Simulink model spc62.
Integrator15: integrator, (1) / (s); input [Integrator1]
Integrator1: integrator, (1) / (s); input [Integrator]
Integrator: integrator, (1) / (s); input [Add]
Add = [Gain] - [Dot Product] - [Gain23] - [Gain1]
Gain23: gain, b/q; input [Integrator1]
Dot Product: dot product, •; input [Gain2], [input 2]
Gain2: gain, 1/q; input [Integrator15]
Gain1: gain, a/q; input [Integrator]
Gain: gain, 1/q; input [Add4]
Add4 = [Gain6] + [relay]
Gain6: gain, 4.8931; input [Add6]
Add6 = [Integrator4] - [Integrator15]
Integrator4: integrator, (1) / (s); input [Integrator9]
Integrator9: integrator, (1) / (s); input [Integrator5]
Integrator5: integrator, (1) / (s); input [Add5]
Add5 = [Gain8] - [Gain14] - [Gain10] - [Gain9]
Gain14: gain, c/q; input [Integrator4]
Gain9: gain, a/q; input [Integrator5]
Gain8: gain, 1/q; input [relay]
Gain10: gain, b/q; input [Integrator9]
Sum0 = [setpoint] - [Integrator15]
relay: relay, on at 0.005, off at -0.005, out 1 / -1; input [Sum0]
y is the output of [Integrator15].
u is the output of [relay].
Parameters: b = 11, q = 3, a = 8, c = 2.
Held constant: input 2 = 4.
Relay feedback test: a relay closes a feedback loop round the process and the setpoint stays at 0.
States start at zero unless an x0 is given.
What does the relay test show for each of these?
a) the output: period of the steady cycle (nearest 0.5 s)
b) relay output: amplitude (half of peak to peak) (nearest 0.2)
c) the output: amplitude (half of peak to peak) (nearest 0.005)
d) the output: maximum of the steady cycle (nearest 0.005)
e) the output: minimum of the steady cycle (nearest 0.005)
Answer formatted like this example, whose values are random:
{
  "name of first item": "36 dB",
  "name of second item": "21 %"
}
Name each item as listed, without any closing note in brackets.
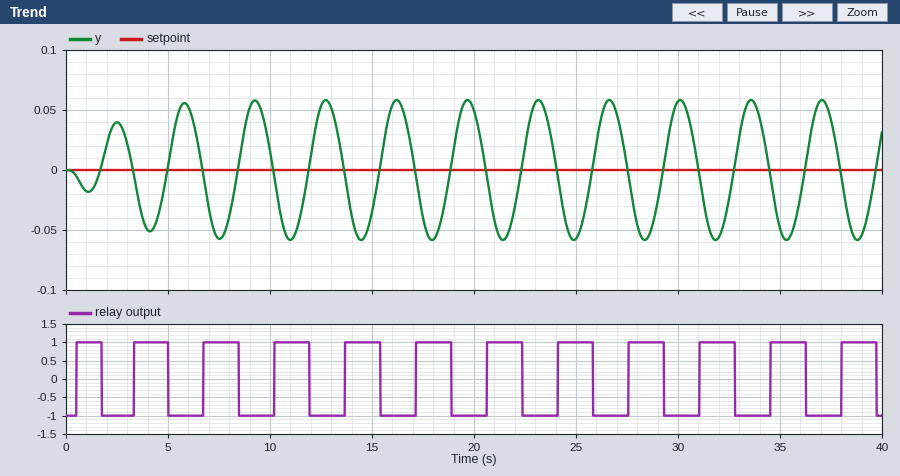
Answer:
{
  "the output: period of the steady cycle": "3.5 s",
  "relay output: amplitude (half of peak to peak)": "1.0",
  "the output: amplitude (half of peak to peak)": "0.060",
  "the output: maximum of the steady cycle": "0.060",
  "the output: minimum of the steady cycle": "-0.060"
}
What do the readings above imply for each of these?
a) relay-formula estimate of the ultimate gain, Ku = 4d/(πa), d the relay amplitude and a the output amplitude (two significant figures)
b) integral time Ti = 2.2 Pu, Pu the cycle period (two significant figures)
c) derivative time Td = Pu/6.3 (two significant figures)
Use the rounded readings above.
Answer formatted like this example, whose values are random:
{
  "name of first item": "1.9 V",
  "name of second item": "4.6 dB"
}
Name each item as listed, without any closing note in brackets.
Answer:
{
  "relay-formula estimate of the ultimate gain, Ku = 4d/(πa), d the relay amplitude and a the output amplitude": "21",
  "integral time Ti = 2.2 Pu, Pu the cycle period": "7.7 s",
  "derivative time Td = Pu/6.3": "0.56 s"
}
